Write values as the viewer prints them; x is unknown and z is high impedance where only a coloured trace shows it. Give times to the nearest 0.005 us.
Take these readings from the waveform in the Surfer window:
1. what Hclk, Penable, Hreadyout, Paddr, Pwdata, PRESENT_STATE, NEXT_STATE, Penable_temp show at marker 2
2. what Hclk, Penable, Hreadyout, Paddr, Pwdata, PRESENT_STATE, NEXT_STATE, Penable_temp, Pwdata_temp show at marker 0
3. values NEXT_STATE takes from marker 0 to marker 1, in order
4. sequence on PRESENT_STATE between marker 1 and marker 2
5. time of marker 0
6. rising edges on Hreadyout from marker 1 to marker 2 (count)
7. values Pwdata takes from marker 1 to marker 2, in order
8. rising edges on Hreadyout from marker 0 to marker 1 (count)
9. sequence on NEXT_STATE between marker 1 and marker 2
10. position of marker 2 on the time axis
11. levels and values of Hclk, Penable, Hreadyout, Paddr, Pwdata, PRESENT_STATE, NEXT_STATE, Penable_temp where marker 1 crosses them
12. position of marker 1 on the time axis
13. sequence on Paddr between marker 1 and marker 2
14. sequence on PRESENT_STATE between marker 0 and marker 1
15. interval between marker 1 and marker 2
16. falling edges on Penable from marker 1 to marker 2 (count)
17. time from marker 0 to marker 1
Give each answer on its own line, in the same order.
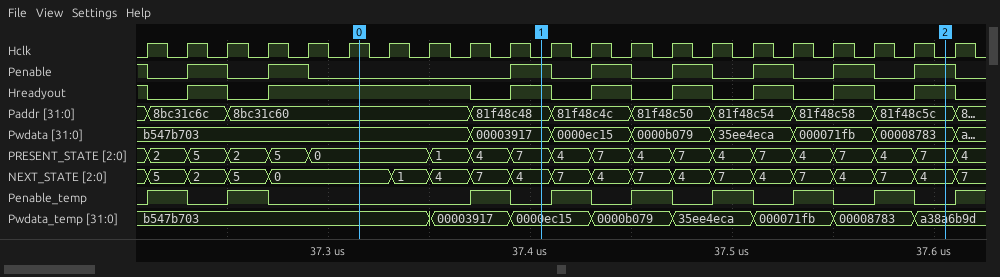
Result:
Hclk=0, Penable=1, Hreadyout=1, Paddr=81f48c5c, Pwdata=00008783, PRESENT_STATE=7, NEXT_STATE=4, Penable_temp=0
Hclk=1, Penable=0, Hreadyout=1, Paddr=8bc31c60, Pwdata=b547b703, PRESENT_STATE=0, NEXT_STATE=0, Penable_temp=0, Pwdata_temp=b547b703
0, 1, 4, 7, 4
7, 4, 7, 4, 7, 4, 7, 4, 7, 4, 7
37.315 us
5
00003917, 0000ec15, 0000b079, 35ee4eca, 000071fb, 00008783
1
4, 7, 4, 7, 4, 7, 4, 7, 4, 7, 4
37.605 us
Hclk=0, Penable=1, Hreadyout=1, Paddr=81f48c48, Pwdata=00003917, PRESENT_STATE=7, NEXT_STATE=4, Penable_temp=0
37.405 us
81f48c48, 81f48c4c, 81f48c50, 81f48c54, 81f48c58, 81f48c5c
0, 1, 4, 7
0.2 us
5
0.09 us
